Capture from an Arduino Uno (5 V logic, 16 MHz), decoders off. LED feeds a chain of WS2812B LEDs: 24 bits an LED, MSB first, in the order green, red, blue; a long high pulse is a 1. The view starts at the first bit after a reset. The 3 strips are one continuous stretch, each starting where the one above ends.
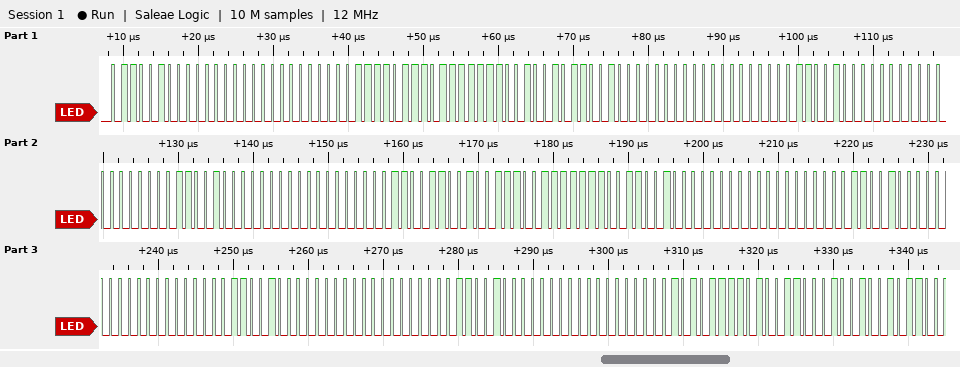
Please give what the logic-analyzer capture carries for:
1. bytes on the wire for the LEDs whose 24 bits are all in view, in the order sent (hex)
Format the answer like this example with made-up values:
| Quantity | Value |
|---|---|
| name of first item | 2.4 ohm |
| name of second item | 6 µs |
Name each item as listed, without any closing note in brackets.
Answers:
| Quantity | Value |
|---|---|
| bytes on the wire for the LEDs whose 24 bits are all in view, in the order sent | 64 00 00 3D DF C9 64 00 00 64 00 00 64 00 00 CC 9C FE 64 00 00 64 00 00 64 00 00 64 00 00 AF 4C 49 |
